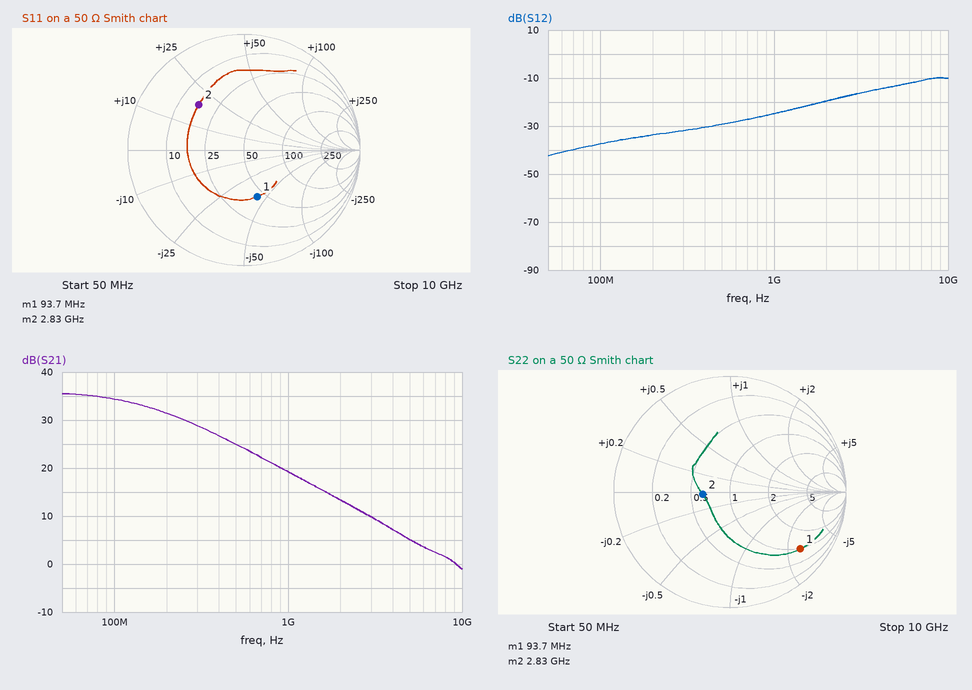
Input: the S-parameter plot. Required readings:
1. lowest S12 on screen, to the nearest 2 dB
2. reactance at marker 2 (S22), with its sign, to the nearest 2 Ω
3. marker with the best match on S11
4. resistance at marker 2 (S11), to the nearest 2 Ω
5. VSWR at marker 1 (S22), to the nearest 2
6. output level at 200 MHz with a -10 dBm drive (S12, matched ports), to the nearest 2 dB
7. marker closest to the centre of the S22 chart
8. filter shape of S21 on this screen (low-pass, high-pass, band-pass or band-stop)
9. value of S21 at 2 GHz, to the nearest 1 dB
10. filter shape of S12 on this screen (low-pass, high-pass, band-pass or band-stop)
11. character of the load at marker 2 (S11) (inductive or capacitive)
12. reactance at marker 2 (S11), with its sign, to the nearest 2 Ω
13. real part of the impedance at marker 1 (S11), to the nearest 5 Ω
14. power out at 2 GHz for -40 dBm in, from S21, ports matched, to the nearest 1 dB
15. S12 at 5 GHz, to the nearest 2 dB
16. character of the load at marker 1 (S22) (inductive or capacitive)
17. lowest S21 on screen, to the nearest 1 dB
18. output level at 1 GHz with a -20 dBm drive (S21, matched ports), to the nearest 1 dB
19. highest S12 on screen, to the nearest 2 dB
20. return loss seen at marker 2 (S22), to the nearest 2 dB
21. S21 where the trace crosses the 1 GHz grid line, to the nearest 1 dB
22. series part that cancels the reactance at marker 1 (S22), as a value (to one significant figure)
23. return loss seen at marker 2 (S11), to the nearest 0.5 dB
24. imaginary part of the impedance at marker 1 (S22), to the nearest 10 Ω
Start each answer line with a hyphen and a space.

- -42 dB
- -2 Ω
- marker 1
- 16 Ω
- 8
- -44 dBm
- marker 2
- low-pass
- 13 dB
- high-pass
- inductive
- +18 Ω
- 45 Ω
- -27 dBm
- -14 dB
- capacitive
- -1 dB
- -1 dBm
- -10 dB
- 12 dB
- 19 dB
- 200 nH
- 5.0 dB
- -120 Ω
